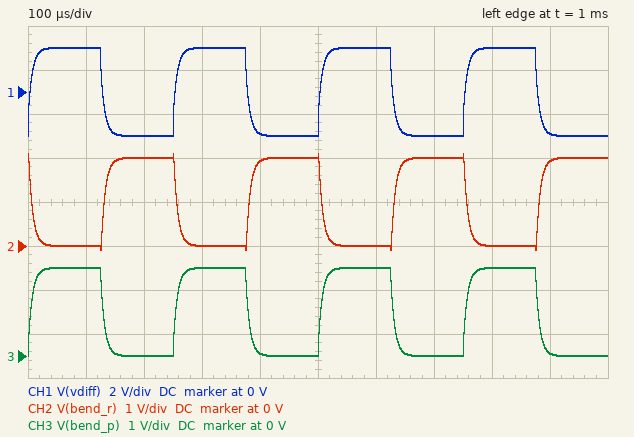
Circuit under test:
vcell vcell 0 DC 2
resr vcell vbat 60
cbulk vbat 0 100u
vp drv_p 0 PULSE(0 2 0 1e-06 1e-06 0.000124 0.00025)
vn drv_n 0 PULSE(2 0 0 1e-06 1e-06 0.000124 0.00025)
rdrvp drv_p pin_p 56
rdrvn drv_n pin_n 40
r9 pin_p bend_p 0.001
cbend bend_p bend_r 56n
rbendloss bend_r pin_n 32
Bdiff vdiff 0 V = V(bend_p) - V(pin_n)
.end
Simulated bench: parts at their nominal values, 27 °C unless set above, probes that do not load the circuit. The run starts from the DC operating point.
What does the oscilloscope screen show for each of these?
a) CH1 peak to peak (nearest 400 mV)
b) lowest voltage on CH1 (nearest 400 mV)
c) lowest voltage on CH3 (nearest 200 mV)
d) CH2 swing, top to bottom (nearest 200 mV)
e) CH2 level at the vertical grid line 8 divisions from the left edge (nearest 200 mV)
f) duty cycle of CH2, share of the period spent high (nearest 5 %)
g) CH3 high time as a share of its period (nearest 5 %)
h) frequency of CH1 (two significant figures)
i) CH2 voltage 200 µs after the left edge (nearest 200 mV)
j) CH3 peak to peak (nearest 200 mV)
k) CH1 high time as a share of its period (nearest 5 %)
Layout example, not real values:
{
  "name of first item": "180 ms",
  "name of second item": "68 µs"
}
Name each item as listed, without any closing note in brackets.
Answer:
{
  "CH1 peak to peak": "4.0 V",
  "lowest voltage on CH1": "-2.0 V",
  "lowest voltage on CH3": "0 V",
  "CH2 swing, top to bottom": "2.2 V",
  "CH2 level at the vertical grid line 8 divisions from the left edge": "0 V",
  "duty cycle of CH2, share of the period spent high": "50 %",
  "CH3 high time as a share of its period": "50 %",
  "frequency of CH1": "4.0 kHz",
  "CH2 voltage 200 µs after the left edge": "2.0 V",
  "CH3 peak to peak": "2.0 V",
  "CH1 high time as a share of its period": "50 %"
}
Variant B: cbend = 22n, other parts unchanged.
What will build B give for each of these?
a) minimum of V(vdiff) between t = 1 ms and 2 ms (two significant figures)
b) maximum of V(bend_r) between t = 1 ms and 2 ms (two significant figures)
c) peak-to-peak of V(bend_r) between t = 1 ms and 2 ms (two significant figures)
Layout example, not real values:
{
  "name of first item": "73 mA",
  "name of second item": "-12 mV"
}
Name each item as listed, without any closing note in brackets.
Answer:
{
  "minimum of V(vdiff) between t = 1 ms and 2 ms": "-2.0 V",
  "maximum of V(bend_r) between t = 1 ms and 2 ms": "2.0 V",
  "peak-to-peak of V(bend_r) between t = 1 ms and 2 ms": "2.1 V"
}
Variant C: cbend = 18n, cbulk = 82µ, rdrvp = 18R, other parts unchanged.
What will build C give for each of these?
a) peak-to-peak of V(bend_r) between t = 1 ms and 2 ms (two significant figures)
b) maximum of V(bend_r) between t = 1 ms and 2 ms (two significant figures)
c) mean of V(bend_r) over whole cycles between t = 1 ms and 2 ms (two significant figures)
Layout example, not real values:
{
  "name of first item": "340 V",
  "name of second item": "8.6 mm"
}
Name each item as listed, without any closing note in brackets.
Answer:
{
  "peak-to-peak of V(bend_r) between t = 1 ms and 2 ms": "2.8 V",
  "maximum of V(bend_r) between t = 1 ms and 2 ms": "2.4 V",
  "mean of V(bend_r) over whole cycles between t = 1 ms and 2 ms": "1.0 V"
}
